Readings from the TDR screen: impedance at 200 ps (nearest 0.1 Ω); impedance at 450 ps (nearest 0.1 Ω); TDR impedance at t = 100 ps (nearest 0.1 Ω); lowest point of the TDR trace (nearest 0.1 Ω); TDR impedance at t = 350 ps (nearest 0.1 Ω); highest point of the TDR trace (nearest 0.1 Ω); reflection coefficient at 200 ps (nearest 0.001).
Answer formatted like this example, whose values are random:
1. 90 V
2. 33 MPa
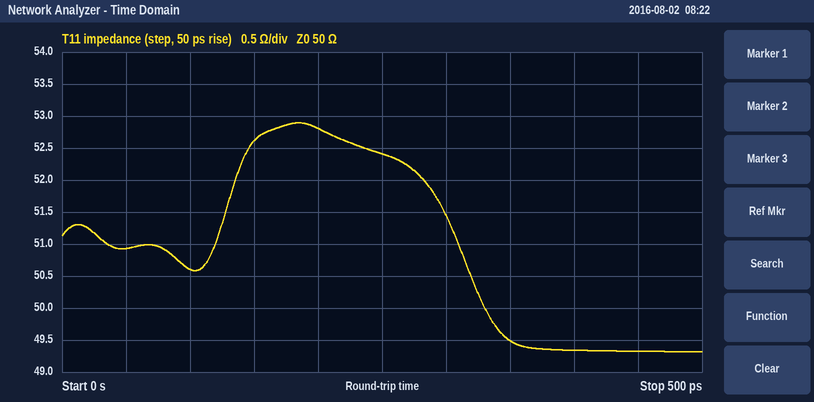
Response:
1. 52.8 Ω
2. 49.3 Ω
3. 50.6 Ω
4. 49.3 Ω
5. 49.5 Ω
6. 52.9 Ω
7. +0.027
